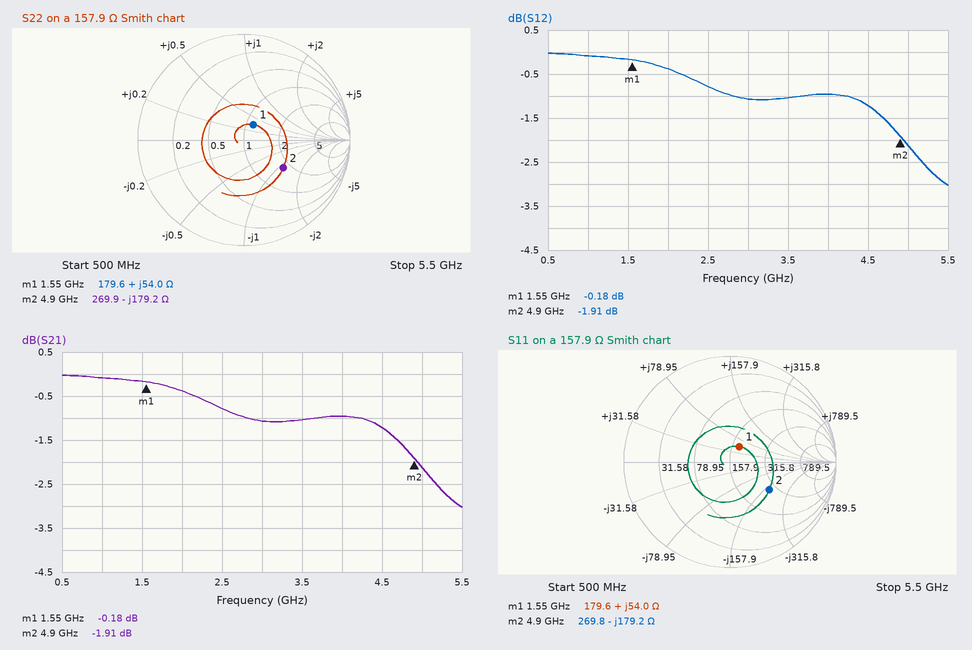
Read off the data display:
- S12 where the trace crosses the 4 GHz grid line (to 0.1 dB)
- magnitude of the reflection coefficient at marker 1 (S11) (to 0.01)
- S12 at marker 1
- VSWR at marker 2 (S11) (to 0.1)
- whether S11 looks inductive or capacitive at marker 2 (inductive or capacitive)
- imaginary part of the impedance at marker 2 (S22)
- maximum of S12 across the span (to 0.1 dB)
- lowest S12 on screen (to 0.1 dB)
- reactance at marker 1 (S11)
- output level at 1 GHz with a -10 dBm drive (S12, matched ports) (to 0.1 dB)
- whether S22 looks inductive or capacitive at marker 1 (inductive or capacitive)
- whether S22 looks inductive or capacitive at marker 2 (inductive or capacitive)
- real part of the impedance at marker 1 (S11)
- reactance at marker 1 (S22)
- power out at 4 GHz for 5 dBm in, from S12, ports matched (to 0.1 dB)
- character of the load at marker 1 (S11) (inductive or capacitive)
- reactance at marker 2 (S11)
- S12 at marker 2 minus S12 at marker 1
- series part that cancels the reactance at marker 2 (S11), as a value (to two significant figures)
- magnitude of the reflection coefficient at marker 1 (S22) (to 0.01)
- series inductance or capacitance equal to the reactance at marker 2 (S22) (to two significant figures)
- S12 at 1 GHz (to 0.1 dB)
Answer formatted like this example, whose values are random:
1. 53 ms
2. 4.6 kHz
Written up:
1. -1.0 dB
2. 0.17
3. -0.18 dB
4. 2.7
5. capacitive
6. -179.2 Ω
7. 0.0 dB
8. -3.0 dB
9. +54.0 Ω
10. -10.1 dBm
11. inductive
12. capacitive
13. 179.6 Ω
14. +54.0 Ω
15. 4.0 dBm
16. inductive
17. -179.2 Ω
18. -1.73 dB
19. 5.8 nH
20. 0.17
21. 180 fF
22. -0.1 dB
